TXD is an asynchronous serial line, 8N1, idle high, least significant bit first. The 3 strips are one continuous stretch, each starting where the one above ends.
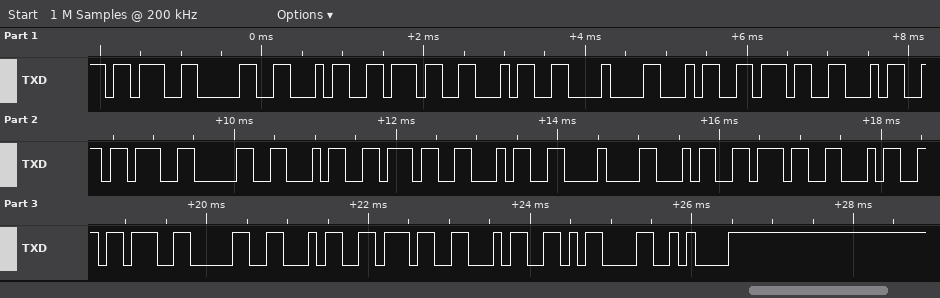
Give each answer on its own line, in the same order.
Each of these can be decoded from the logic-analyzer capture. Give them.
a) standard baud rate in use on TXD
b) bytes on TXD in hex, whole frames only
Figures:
9600 baud
3B 30 34 37 34 08 34 37 34 3B 30 34 37 34 08 34 37 34 3B 30 34 37 34 0D 0A
